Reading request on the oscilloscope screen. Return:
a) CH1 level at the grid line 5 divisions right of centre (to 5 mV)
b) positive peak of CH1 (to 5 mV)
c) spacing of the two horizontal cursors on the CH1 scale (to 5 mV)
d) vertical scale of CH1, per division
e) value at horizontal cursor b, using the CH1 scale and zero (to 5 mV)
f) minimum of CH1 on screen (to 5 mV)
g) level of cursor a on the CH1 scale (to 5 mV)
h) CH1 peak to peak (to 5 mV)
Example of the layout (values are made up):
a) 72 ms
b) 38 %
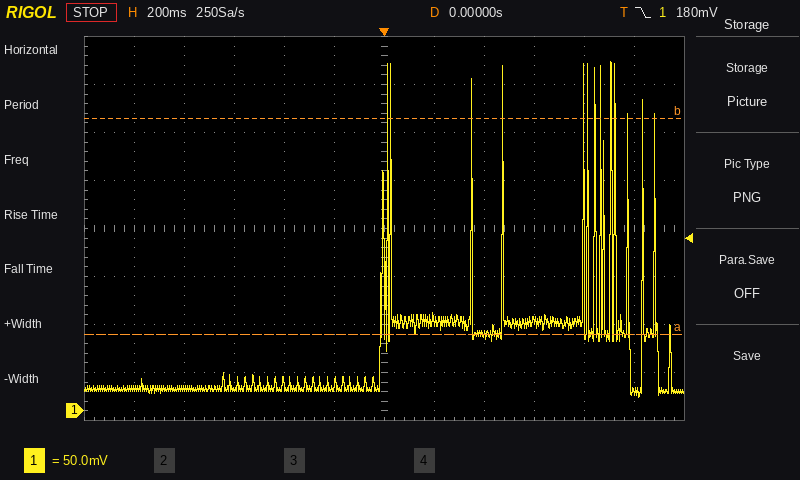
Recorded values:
a) 20 mV
b) 365 mV
c) 225 mV
d) 50 mV
e) 305 mV
f) 15 mV
g) 80 mV
h) 350 mV
